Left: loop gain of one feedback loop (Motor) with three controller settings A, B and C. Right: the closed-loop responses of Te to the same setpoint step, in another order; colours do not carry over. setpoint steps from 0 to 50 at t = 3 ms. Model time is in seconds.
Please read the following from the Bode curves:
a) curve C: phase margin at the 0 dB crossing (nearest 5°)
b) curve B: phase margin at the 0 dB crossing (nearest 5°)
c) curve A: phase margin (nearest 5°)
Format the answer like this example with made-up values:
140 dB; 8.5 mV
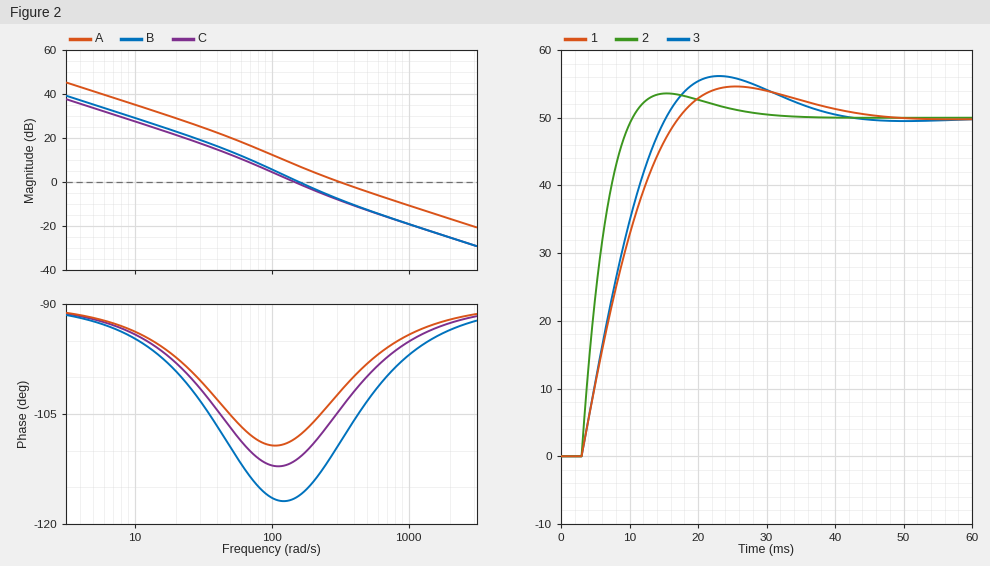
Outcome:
70°; 65°; 80°
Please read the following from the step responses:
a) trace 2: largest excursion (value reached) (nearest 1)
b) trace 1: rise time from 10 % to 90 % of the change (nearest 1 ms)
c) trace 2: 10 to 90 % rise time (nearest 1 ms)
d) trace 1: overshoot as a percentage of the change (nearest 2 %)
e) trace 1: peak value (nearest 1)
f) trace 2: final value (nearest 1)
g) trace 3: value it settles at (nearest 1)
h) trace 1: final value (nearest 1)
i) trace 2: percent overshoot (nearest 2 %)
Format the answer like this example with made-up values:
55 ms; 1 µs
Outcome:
54; 10 ms; 5 ms; 10 %; 55; 50; 50; 50; 8 %
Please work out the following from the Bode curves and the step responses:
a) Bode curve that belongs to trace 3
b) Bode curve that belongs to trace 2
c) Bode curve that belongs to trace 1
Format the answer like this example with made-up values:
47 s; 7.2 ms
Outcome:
B; A; C
